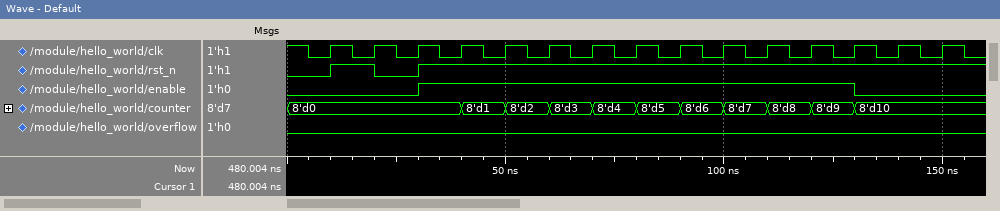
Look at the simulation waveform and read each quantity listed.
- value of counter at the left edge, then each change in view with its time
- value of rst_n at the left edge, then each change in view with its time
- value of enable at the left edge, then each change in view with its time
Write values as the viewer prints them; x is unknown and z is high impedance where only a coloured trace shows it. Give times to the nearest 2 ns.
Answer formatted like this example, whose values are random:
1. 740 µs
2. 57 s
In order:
1. 8'd0, 8'd1 at 40 ns, 8'd2 at 50 ns, 8'd3 at 60 ns, 8'd4 at 70 ns, 8'd5 at 80 ns, 8'd6 at 90 ns, 8'd7 at 100 ns, 8'd8 at 110 ns, 8'd9 at 120 ns, 8'd10 at 130 ns
2. 0, 1 at 10 ns, 0 at 20 ns, 1 at 30 ns
3. 0, 1 at 30 ns, 0 at 130 ns
